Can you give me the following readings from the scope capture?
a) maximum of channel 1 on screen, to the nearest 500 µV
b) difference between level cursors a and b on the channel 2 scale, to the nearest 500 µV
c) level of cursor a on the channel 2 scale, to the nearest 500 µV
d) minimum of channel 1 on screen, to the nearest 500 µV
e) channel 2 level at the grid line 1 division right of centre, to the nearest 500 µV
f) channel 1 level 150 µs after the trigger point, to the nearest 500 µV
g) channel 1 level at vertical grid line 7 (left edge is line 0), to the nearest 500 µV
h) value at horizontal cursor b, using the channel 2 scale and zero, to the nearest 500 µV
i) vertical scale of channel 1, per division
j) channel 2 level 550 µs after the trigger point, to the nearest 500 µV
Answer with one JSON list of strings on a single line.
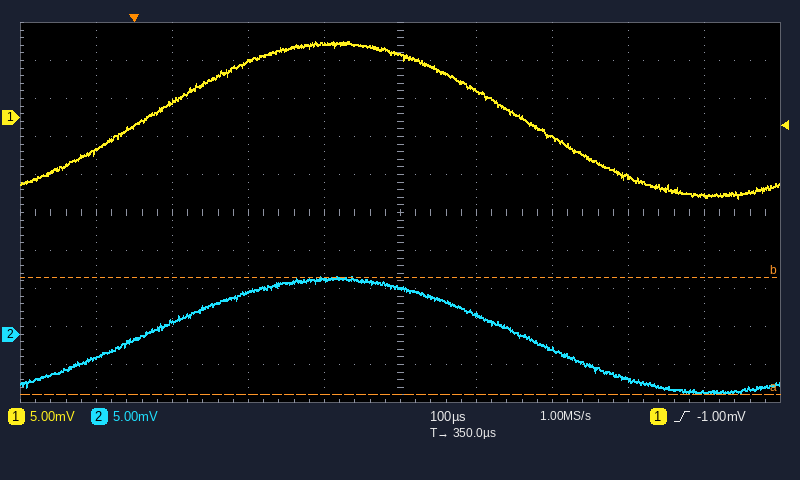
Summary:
["10.0 mV", "15.5 mV", "-8.0 mV", "-10.5 mV", "2.5 mV", "7.5 mV", "-2.5 mV", "7.5 mV", "5 mV", "-2.0 mV"]
